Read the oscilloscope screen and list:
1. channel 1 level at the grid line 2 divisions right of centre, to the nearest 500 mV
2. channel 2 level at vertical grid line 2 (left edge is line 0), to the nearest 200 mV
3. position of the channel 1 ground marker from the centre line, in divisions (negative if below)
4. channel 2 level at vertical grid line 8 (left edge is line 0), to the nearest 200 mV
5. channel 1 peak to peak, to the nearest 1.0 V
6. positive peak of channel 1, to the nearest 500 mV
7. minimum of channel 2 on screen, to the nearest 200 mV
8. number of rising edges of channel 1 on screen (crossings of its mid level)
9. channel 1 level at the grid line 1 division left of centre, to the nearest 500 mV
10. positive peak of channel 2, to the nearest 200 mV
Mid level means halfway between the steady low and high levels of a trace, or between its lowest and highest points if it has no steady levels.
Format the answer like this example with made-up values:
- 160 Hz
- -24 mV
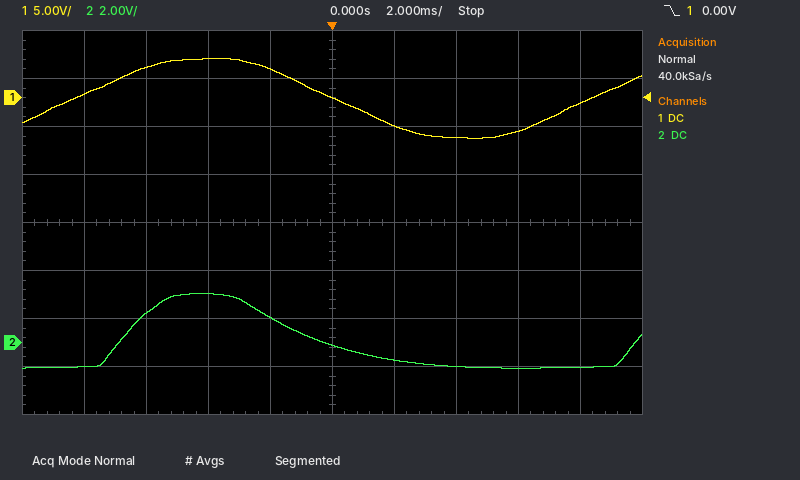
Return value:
- -4.0 V
- 1.2 V
- +2.6 div
- -1.0 V
- 8.0 V
- 4.0 V
- -1.0 V
- 2
- 3.0 V
- 2.0 V
